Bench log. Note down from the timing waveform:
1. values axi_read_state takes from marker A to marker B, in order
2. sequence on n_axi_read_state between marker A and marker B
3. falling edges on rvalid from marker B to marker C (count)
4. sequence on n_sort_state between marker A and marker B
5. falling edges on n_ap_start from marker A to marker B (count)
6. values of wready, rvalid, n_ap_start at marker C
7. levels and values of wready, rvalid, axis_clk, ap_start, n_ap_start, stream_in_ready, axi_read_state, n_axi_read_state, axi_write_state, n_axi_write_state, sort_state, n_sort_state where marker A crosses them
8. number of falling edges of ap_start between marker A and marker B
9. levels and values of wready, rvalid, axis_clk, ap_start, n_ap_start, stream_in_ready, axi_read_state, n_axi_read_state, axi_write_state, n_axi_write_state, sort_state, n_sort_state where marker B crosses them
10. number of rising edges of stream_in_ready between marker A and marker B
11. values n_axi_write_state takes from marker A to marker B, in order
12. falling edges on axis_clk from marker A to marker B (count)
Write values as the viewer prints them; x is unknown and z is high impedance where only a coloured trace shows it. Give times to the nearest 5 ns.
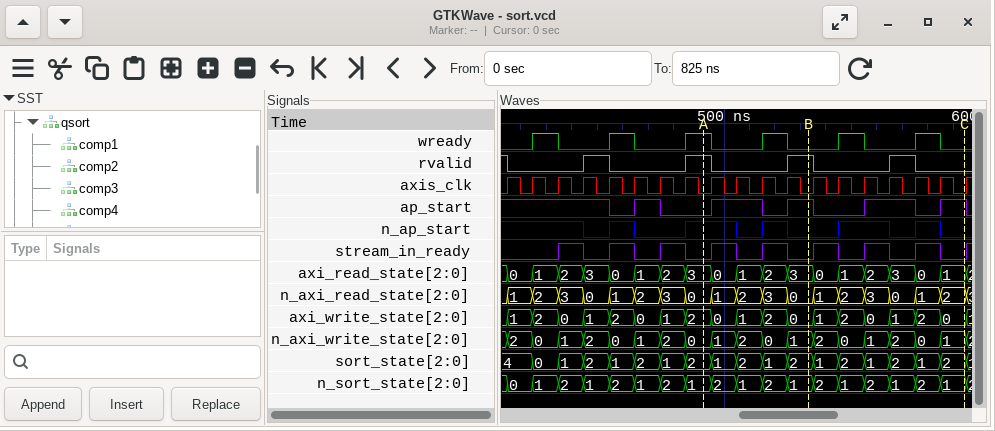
3, 0, 1, 2, 3
0, 1, 2, 3, 0
2
1, 2, 1, 2, 1
2
wready=0, rvalid=0, n_ap_start=0
wready=1, rvalid=1, axis_clk=0, ap_start=0, n_ap_start=1, stream_in_ready=0, axi_read_state=3, n_axi_read_state=0, axi_write_state=2, n_axi_write_state=0, sort_state=2, n_sort_state=1
1
wready=0, rvalid=1, axis_clk=0, ap_start=1, n_ap_start=0, stream_in_ready=0, axi_read_state=3, n_axi_read_state=0, axi_write_state=0, n_axi_write_state=1, sort_state=2, n_sort_state=1
2
0, 1, 2, 0, 1
4
